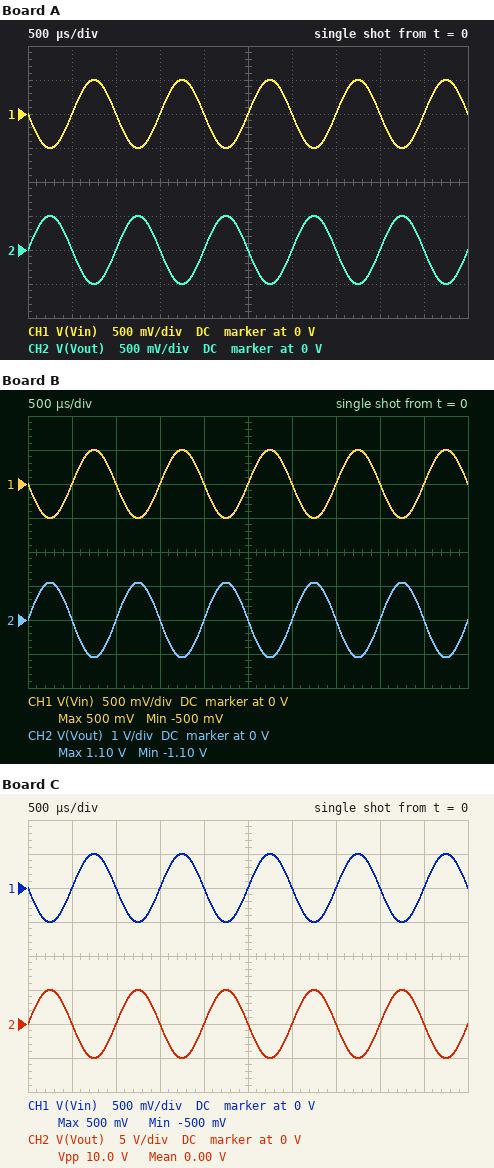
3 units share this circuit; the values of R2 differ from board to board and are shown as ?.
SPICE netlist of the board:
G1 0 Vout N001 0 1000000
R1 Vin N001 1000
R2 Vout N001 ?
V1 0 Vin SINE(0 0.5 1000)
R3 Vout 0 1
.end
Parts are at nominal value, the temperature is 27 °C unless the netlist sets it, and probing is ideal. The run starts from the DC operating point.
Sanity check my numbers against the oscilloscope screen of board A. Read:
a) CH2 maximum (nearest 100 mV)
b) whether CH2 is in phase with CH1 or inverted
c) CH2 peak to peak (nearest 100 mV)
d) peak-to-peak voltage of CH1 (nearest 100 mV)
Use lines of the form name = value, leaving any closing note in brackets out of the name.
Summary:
CH2 maximum = 500 mV
whether CH2 is in phase with CH1 or inverted = inverted
CH2 peak to peak = 1.0 V
peak-to-peak voltage of CH1 = 1.0 V
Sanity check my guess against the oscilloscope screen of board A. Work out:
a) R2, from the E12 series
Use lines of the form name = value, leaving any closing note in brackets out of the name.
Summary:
R2, from the E12 series = 1 kΩ
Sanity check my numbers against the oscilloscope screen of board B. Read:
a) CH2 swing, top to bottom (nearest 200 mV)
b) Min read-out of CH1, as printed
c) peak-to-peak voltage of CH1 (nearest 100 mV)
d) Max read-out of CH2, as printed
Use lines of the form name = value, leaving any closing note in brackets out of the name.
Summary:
CH2 swing, top to bottom = 2.2 V
Min read-out of CH1, as printed = -500 mV
peak-to-peak voltage of CH1 = 1.0 V
Max read-out of CH2, as printed = 1.10 V
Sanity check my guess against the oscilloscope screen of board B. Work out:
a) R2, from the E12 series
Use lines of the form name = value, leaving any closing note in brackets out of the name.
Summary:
R2, from the E12 series = 2.2 kΩ
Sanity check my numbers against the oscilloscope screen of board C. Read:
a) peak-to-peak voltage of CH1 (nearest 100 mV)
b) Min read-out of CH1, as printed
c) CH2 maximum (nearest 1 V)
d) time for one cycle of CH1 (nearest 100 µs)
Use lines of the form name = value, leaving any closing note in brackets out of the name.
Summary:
peak-to-peak voltage of CH1 = 1.0 V
Min read-out of CH1, as printed = -500 mV
CH2 maximum = 5 V
time for one cycle of CH1 = 1.0 ms
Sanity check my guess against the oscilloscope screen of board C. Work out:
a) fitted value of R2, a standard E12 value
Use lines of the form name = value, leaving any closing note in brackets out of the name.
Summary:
fitted value of R2, a standard E12 value = 10 kΩ
